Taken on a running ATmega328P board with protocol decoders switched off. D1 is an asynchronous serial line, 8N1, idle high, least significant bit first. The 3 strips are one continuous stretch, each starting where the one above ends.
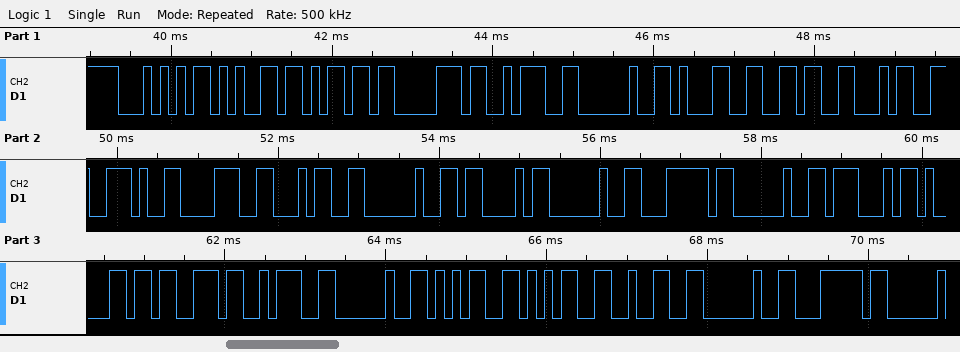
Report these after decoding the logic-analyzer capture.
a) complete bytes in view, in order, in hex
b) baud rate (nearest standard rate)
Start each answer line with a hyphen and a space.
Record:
- 54 65 6D 70 3A 20 31 36 34 2E 38 34 20 43 20 7C 20 47 61 73 3A 20 35 35 32 20 7C
- 9600 baud
